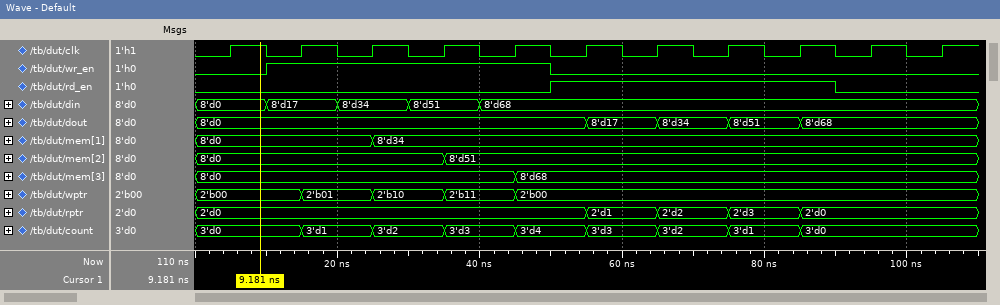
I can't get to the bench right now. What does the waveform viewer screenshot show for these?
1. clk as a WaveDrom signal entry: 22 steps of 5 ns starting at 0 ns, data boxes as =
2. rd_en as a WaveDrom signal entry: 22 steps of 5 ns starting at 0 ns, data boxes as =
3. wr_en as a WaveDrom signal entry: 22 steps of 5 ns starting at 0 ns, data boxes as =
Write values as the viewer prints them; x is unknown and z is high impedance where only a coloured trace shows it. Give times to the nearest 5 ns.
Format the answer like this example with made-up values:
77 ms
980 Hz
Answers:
{name: 'clk', wave: '0101010101010101010101'}
{name: 'rd_en', wave: '0.........1.......0...'}
{name: 'wr_en', wave: '0.1.......0...........'}
